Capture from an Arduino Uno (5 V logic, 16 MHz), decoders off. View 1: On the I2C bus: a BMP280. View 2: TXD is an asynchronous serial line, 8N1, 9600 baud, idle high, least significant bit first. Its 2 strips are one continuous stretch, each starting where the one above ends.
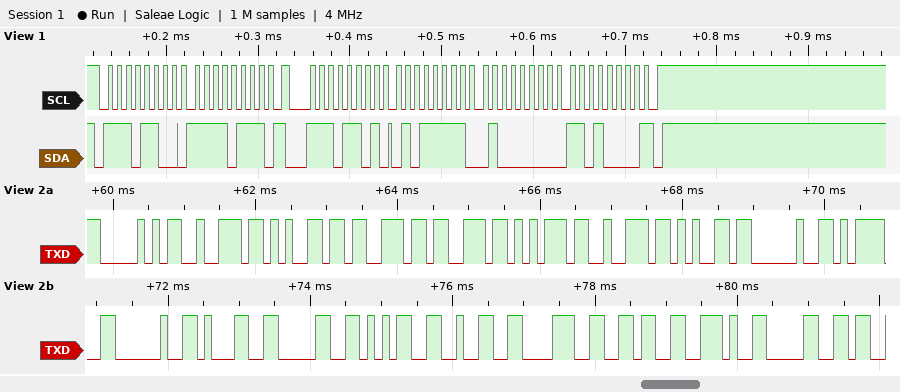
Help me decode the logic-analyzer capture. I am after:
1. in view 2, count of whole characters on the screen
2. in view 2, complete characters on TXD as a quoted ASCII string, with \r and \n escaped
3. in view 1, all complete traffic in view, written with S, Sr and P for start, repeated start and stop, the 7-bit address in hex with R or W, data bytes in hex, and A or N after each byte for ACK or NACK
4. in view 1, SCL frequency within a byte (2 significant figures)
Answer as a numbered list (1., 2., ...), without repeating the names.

1. 19
2. "Pressure = 105286.0"
3. S 76W A F7 A Sr 76R A 5F A 40 A D0 N P
4. 100 kHz
